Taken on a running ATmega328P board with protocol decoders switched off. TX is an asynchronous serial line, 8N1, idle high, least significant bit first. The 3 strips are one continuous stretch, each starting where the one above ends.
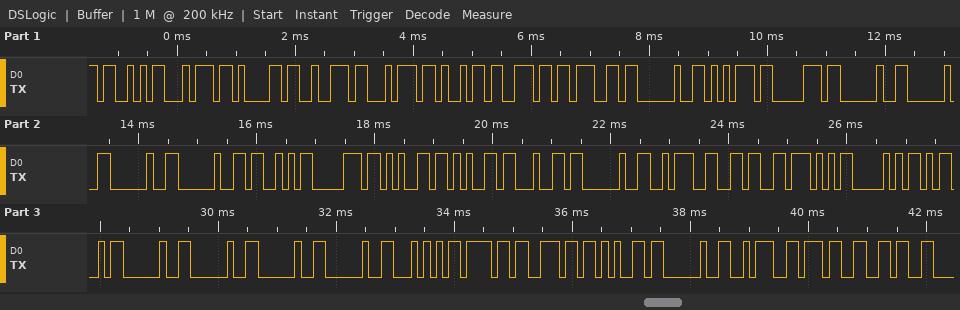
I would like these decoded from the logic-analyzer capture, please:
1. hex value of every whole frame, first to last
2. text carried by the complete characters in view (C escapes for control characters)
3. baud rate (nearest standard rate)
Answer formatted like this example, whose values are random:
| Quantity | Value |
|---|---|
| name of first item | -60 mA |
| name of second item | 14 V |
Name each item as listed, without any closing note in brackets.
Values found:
| Quantity | Value |
|---|---|
| hex value of every whole frame, first to last | 53 74 61 72 74 69 6E 67 20 75 70 20 20 20 20 53 70 65 65 64 20 3A 36 57 50 4D 20 20 20 20 54 6F 6E 65 20 3A 37 36 |
| text carried by the complete characters in view | "Starting up    Speed :6WPM    Tone :76" |
| baud rate | 9600 baud |
